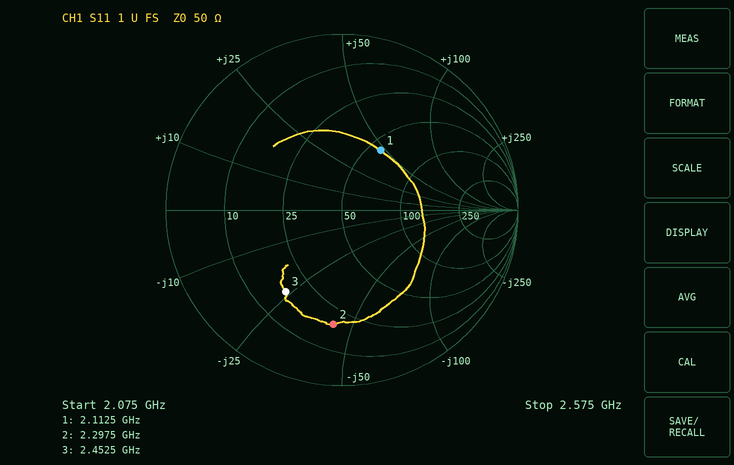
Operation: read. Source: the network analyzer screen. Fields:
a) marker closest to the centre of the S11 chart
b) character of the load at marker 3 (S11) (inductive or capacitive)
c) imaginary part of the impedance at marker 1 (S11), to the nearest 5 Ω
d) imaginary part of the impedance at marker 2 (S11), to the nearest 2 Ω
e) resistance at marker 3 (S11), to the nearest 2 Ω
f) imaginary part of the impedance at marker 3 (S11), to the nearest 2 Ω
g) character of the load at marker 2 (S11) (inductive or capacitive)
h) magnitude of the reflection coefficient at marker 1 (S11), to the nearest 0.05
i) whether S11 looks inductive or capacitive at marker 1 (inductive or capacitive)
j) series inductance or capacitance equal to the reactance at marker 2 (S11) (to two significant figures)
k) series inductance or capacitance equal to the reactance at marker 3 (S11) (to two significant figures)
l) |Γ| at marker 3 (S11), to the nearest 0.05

marker 1
capacitive
+45 Ω
-42 Ω
18 Ω
-24 Ω
capacitive
0.40
inductive
1.6 pF
2.7 pF
0.55
